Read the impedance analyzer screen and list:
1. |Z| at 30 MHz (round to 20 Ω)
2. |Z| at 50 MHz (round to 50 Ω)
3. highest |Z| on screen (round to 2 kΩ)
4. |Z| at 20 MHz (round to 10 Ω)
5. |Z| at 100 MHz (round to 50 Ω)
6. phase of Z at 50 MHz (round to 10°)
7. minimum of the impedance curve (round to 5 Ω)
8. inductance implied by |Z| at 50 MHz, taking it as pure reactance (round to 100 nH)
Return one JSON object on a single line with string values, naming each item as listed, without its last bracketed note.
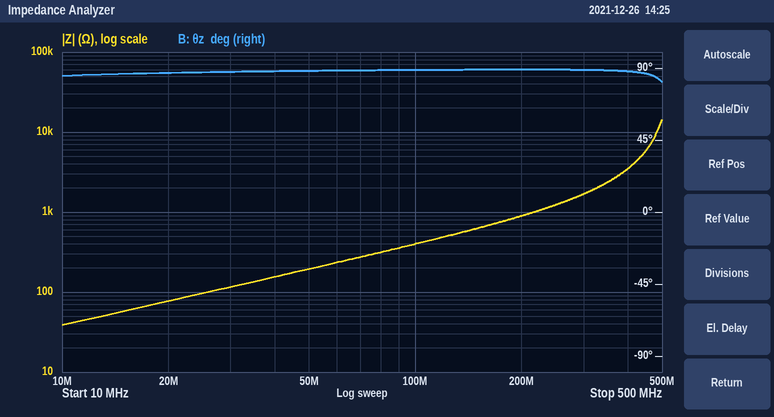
{"|Z| at 30 MHz": "120 Ω", "|Z| at 50 MHz": "200 Ω", "highest |Z| on screen": "14 kΩ", "|Z| at 20 MHz": "80 Ω", "|Z| at 100 MHz": "400 Ω", "phase of Z at 50 MHz": "90°", "minimum of the impedance curve": "40 Ω", "inductance implied by |Z| at 50 MHz, taking it as pure reactance": "600 nH"}
